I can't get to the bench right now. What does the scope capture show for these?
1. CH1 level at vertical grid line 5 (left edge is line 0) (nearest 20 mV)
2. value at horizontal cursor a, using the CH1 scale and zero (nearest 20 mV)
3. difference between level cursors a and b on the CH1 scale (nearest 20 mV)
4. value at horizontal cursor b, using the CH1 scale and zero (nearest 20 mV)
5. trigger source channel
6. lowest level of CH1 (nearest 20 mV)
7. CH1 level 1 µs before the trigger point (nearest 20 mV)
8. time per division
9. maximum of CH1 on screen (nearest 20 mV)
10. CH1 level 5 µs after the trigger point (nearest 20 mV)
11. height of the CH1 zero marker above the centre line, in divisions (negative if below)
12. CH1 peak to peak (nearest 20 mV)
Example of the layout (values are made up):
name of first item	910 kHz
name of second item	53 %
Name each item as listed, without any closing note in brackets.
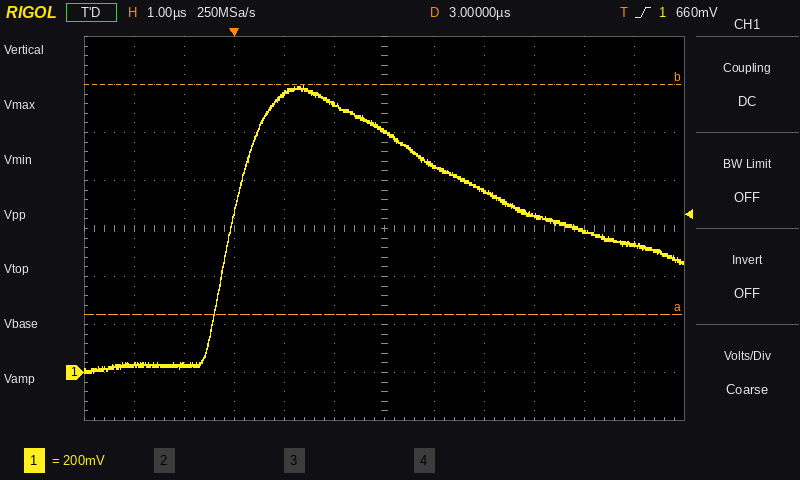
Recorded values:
CH1 level at vertical grid line 5 (left edge is line 0)	1.12 V
value at horizontal cursor a, using the CH1 scale and zero	240 mV
difference between level cursors a and b on the CH1 scale	960 mV
value at horizontal cursor b, using the CH1 scale and zero	1.20 V
trigger source channel	CH1
lowest level of CH1	0 mV
CH1 level 1 µs before the trigger point	40 mV
time per division	1 µs
maximum of CH1 on screen	1.20 V
CH1 level 5 µs after the trigger point	760 mV
height of the CH1 zero marker above the centre line, in divisions	-3.0 div
CH1 peak to peak	1.20 V
